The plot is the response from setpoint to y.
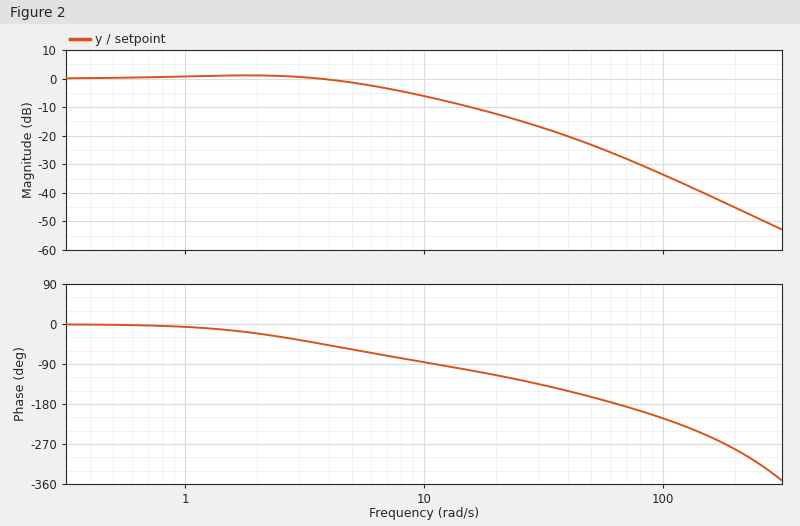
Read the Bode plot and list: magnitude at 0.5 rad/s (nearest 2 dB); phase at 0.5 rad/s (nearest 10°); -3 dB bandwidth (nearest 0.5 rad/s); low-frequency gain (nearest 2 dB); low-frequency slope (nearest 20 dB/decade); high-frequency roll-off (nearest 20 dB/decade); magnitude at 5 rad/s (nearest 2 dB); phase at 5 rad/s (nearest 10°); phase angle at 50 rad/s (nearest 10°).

0 dB
0°
6.5 rad/s
0 dB
0 dB/decade
-40 dB/decade
-2 dB
-60°
-160°
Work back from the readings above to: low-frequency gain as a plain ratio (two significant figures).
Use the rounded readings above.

1.0
